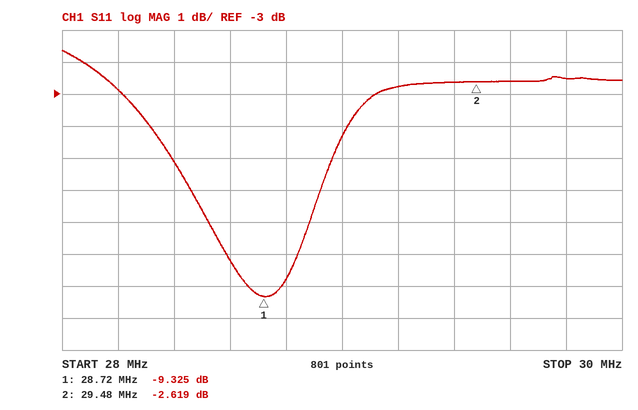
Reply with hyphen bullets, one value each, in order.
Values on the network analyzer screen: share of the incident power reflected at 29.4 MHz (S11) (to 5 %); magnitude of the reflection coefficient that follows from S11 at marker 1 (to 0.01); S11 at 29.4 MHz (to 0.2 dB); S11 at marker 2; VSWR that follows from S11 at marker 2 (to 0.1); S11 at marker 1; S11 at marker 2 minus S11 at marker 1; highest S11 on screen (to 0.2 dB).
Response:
- 55 %
- 0.34
- -2.6 dB
- -2.619 dB
- 6.7
- -9.325 dB
- 6.706 dB
- -1.6 dB
